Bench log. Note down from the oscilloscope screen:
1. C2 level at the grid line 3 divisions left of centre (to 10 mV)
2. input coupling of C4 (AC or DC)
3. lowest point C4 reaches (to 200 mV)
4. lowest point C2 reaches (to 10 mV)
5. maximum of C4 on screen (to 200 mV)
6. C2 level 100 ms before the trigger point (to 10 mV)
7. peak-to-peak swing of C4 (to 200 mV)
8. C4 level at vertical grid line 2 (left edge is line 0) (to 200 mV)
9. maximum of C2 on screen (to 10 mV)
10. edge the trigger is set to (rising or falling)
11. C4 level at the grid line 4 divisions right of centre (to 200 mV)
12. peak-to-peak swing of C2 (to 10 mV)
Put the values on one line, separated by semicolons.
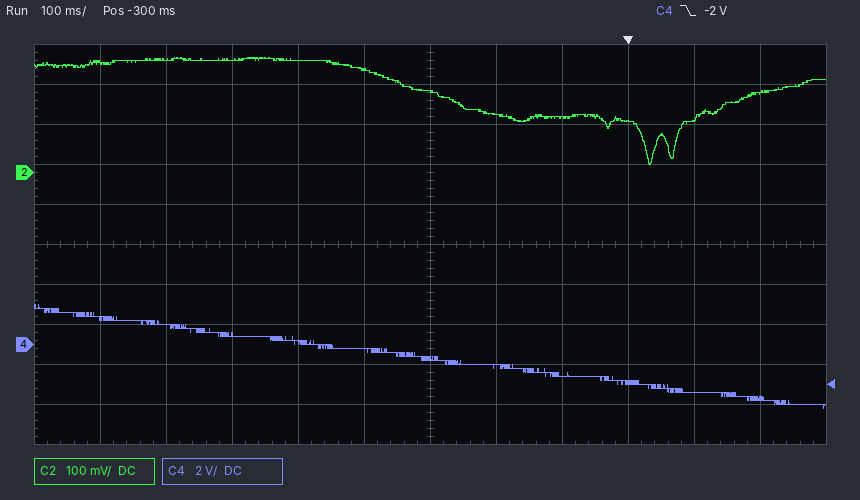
280 mV; DC; -3.2 V; 20 mV; 2.0 V; 140 mV; 5.2 V; 1.0 V; 290 mV; falling; -2.4 V; 270 mV
